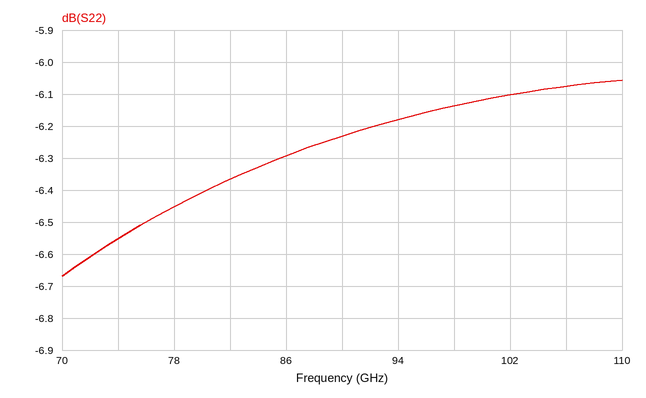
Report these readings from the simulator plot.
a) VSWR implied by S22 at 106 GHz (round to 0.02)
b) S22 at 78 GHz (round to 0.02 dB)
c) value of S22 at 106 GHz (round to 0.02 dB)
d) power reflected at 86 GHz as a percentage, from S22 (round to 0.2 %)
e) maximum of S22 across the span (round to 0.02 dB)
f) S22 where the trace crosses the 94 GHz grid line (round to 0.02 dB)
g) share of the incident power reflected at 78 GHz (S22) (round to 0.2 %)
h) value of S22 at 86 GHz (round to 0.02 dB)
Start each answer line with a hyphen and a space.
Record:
- 2.98
- -6.46 dB
- -6.08 dB
- 23.4 %
- -6.06 dB
- -6.18 dB
- 22.6 %
- -6.30 dB
